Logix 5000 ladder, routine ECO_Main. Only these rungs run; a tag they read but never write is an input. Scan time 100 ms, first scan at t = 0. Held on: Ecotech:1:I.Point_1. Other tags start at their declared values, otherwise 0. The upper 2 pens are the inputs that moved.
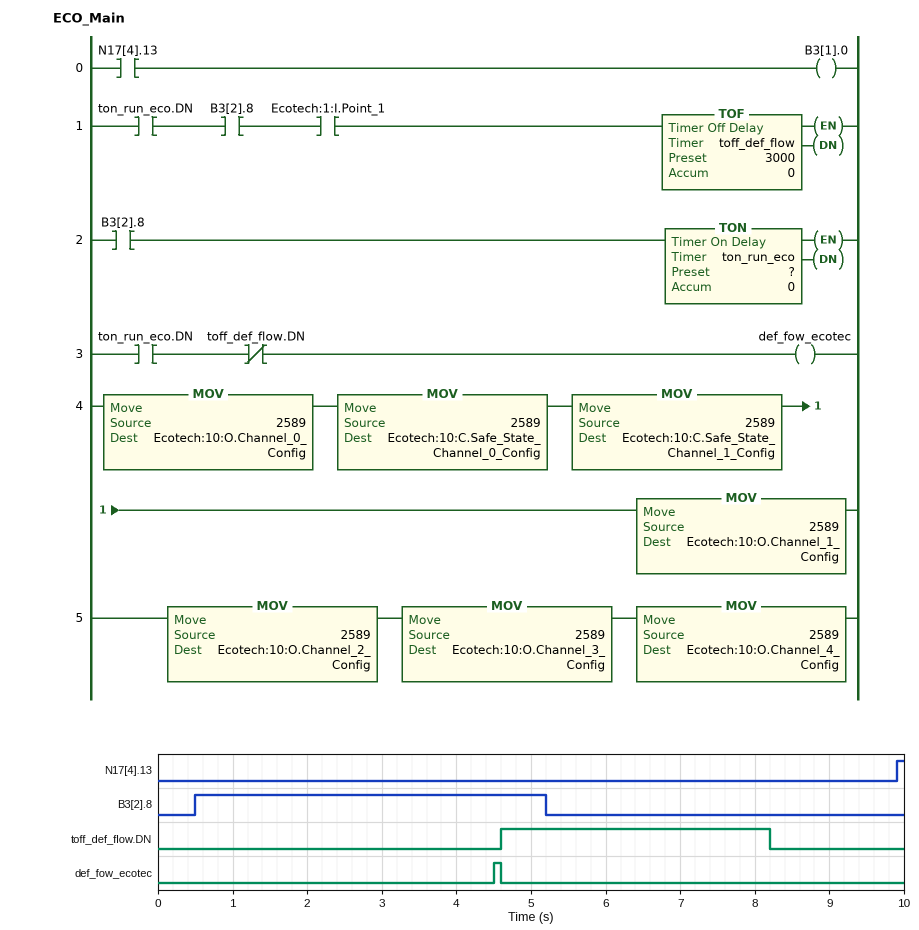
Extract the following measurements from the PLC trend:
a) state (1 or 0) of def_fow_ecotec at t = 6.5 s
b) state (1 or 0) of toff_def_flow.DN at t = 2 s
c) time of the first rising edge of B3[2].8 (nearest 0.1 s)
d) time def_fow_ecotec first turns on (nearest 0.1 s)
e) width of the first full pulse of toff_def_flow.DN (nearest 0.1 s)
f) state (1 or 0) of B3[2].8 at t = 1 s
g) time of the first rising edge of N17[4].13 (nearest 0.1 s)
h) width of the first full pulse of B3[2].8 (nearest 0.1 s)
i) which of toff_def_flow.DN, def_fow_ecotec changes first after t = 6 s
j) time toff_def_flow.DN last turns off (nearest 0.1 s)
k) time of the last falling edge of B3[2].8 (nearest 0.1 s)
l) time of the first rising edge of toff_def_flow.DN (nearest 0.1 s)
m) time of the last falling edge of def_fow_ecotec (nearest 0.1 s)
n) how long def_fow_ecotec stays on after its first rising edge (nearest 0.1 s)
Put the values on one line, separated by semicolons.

0; 0; 0.5 s; 4.5 s; 3.6 s; 1; 9.9 s; 4.7 s; toff_def_flow.DN; 8.2 s; 5.2 s; 4.6 s; 4.6 s; 0.1 s
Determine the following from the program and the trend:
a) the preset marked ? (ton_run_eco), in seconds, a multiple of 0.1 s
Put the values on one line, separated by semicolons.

4.0 s
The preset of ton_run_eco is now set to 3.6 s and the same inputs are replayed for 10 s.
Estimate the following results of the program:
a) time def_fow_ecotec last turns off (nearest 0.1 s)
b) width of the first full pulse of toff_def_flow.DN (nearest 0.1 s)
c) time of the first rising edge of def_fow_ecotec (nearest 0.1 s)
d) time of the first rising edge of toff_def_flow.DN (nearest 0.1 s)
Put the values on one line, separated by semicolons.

4.2 s; 4.0 s; 4.1 s; 4.2 s
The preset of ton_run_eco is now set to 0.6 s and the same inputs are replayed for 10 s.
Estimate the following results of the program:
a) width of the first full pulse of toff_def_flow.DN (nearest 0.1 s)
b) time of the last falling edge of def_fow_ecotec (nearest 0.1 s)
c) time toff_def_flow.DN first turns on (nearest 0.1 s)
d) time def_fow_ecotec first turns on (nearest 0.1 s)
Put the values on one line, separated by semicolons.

7.0 s; 1.2 s; 1.2 s; 1.1 s
